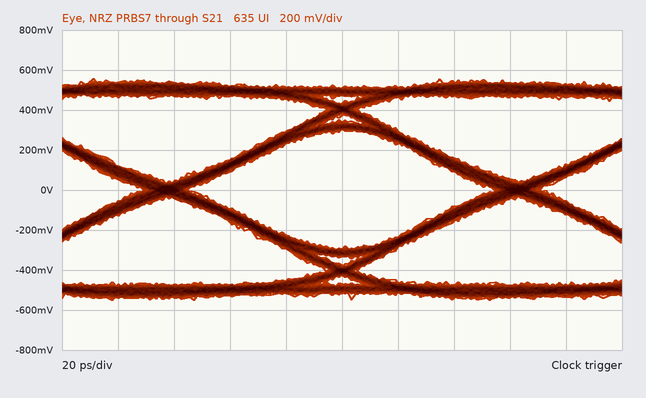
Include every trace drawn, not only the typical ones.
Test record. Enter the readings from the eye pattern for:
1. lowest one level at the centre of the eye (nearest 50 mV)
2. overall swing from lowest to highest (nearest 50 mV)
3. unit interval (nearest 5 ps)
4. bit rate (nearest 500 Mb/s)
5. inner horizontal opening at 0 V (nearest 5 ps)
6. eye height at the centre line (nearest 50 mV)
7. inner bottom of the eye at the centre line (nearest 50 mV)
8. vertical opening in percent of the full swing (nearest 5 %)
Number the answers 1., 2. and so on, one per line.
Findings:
1. 300 mV
2. 1.10 V
3. 125 ps
4. 8.0 Gb/s
5. 110 ps
6. 600 mV
7. -300 mV
8. 55 %
